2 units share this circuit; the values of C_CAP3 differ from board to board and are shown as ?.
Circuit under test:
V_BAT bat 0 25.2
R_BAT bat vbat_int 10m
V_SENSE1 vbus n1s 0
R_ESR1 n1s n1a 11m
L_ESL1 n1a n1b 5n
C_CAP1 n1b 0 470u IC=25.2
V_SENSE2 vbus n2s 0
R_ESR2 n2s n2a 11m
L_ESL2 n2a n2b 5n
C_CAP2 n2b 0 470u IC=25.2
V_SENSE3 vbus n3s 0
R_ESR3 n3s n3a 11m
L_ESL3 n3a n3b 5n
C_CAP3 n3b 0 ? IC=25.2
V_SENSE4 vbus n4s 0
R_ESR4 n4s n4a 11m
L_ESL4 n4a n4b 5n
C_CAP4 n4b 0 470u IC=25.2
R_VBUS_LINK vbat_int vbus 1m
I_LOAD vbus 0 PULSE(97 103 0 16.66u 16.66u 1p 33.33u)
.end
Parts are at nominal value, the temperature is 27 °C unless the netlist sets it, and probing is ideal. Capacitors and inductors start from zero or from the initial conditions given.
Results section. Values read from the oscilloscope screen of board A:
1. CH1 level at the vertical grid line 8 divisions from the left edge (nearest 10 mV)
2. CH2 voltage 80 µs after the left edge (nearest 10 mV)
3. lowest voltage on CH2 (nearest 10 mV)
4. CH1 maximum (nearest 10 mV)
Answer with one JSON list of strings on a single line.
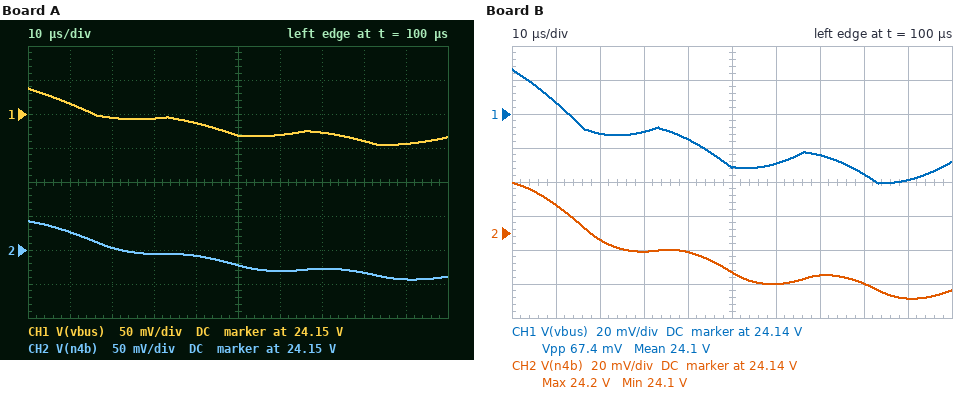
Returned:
["24.11 V", "24.12 V", "24.11 V", "24.19 V"]
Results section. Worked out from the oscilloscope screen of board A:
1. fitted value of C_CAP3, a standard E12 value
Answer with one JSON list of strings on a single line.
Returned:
["1.5 mF"]
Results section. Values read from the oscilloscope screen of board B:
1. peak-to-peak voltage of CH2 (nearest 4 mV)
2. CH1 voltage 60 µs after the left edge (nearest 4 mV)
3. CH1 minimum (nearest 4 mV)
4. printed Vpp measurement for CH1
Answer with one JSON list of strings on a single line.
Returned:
["68 mV", "24.112 V", "24.100 V", "67.4 mV"]
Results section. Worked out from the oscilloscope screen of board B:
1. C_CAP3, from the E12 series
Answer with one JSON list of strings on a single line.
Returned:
["1.2 mF"]
